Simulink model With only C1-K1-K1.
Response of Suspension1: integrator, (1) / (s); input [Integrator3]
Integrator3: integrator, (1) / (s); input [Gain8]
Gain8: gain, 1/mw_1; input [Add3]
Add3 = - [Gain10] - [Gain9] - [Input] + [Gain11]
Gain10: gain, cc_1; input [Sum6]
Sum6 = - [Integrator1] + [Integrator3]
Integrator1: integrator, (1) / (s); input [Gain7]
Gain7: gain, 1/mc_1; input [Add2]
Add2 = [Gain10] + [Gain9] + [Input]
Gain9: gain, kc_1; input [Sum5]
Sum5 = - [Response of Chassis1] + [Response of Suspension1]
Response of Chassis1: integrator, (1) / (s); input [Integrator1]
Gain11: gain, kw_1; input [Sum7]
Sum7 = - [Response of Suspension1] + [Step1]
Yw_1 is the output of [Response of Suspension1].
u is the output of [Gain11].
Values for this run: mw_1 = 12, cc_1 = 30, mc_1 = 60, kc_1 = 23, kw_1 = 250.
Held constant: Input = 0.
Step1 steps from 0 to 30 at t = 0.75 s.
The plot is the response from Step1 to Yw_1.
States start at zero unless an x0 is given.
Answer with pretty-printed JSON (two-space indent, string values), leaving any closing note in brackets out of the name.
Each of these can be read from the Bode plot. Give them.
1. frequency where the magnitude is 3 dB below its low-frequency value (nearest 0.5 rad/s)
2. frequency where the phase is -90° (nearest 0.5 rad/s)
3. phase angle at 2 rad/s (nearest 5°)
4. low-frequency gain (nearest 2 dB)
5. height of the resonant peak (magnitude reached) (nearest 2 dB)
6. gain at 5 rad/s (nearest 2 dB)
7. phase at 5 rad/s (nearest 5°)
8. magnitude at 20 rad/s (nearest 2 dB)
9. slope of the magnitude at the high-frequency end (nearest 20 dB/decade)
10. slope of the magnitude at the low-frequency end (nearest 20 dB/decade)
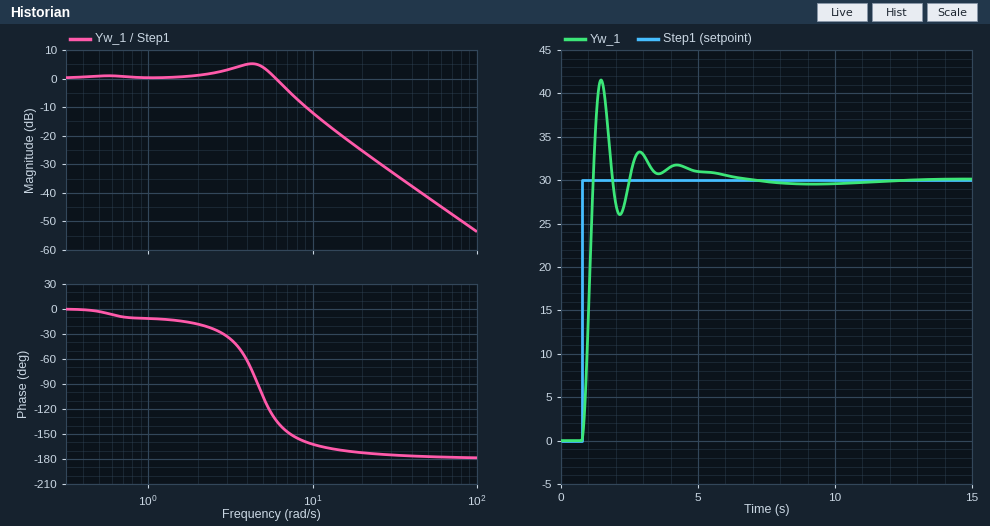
{
  "frequency where the magnitude is 3 dB below its low-frequency value": "6.5 rad/s",
  "frequency where the phase is -90°": "4.5 rad/s",
  "phase angle at 2 rad/s": "-20°",
  "low-frequency gain": "0 dB",
  "height of the resonant peak (magnitude reached)": "6 dB",
  "gain at 5 rad/s": "4 dB",
  "phase at 5 rad/s": "-105°",
  "magnitude at 20 rad/s": "-26 dB",
  "slope of the magnitude at the high-frequency end": "-40 dB/decade",
  "slope of the magnitude at the low-frequency end": "0 dB/decade"
}
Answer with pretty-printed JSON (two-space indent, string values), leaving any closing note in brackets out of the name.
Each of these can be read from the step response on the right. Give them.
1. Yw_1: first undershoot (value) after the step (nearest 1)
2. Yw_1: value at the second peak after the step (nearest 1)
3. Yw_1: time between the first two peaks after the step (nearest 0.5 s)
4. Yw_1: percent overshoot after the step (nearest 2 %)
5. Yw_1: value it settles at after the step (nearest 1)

{
  "Yw_1: first undershoot (value) after the step": "26",
  "Yw_1: value at the second peak after the step": "33",
  "Yw_1: time between the first two peaks after the step": "1.5 s",
  "Yw_1: percent overshoot after the step": "38 %",
  "Yw_1: value it settles at after the step": "30"
}
